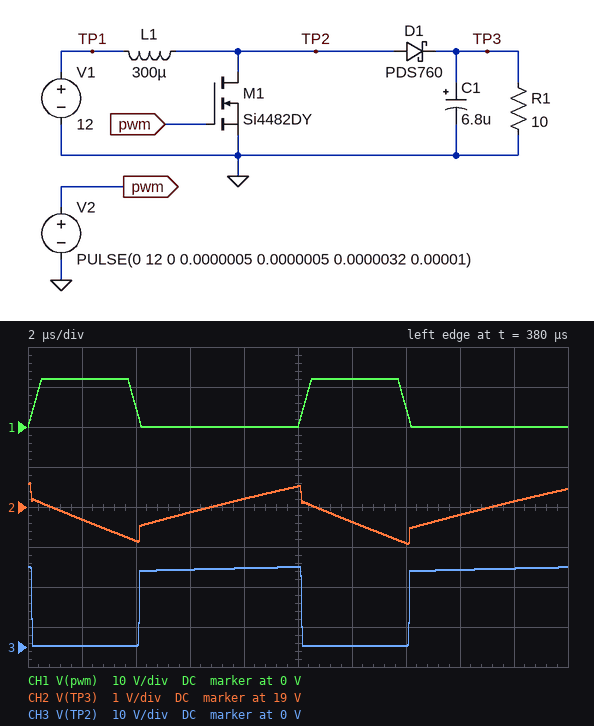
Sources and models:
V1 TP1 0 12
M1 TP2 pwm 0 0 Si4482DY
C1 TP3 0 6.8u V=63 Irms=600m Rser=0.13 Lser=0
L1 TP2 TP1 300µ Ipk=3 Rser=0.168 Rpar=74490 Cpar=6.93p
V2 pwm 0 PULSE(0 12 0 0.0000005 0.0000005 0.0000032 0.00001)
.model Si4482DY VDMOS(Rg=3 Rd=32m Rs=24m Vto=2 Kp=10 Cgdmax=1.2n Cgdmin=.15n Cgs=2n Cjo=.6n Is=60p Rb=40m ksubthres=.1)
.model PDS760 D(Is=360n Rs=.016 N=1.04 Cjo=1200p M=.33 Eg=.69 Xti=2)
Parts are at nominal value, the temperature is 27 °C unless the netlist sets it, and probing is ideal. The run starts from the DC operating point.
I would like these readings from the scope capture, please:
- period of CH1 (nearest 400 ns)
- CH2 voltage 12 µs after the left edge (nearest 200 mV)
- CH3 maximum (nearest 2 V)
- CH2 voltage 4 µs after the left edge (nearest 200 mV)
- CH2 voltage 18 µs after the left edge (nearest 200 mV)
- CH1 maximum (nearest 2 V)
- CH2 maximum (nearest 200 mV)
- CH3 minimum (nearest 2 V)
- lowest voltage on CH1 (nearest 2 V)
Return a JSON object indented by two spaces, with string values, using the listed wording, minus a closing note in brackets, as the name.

{
  "period of CH1": "10.0 µs",
  "CH2 voltage 12 µs after the left edge": "18.6 V",
  "CH3 maximum": "20 V",
  "CH2 voltage 4 µs after the left edge": "18.2 V",
  "CH2 voltage 18 µs after the left edge": "19.2 V",
  "CH1 maximum": "12 V",
  "CH2 maximum": "19.6 V",
  "CH3 minimum": "0 V",
  "lowest voltage on CH1": "0 V"
}
